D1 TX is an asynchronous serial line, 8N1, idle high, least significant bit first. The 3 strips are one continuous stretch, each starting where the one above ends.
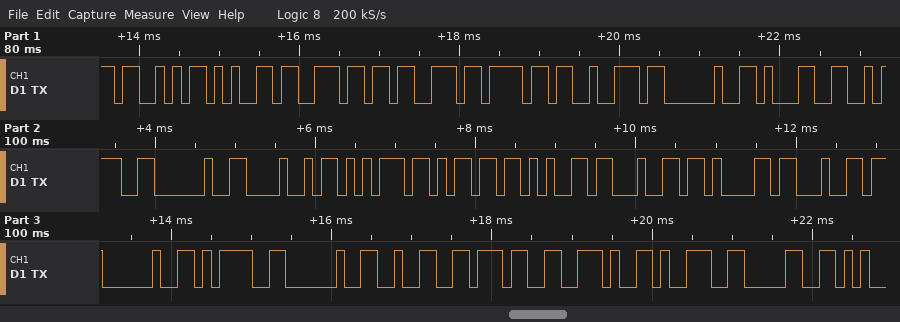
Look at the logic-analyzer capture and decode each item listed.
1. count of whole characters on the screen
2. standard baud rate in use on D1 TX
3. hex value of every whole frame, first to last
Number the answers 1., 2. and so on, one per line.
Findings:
1. 25
2. 9600 baud
3. 53 65 6E 73 6F 72 20 31 3A 20 48 75 6D 65 64 61 64 20 3D 20 32 37 2E 39 30
